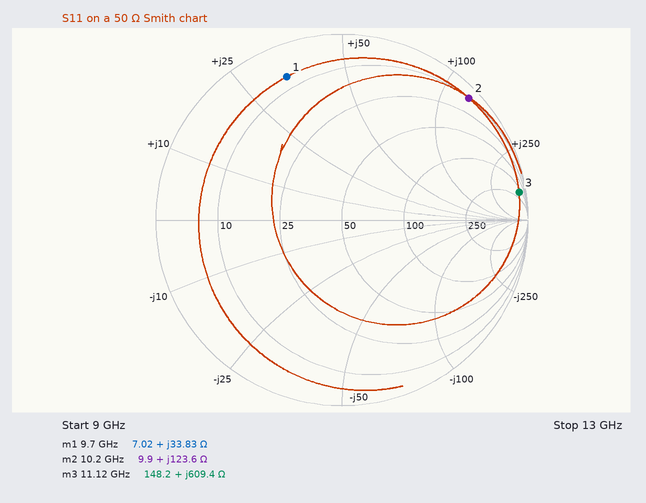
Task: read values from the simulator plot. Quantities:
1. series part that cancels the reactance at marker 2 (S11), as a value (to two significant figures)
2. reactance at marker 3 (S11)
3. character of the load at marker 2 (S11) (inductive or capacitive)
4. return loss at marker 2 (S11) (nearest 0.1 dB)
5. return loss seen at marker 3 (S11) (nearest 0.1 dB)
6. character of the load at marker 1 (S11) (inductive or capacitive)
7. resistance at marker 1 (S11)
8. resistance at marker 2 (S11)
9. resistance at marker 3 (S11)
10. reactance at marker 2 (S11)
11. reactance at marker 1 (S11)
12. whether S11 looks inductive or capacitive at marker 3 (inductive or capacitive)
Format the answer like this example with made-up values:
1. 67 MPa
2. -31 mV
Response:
1. 130 fF
2. +609.4 Ω
3. inductive
4. 0.5 dB
5. 0.3 dB
6. inductive
7. 7.02 Ω
8. 9.9 Ω
9. 148.2 Ω
10. +123.6 Ω
11. +33.83 Ω
12. inductive
